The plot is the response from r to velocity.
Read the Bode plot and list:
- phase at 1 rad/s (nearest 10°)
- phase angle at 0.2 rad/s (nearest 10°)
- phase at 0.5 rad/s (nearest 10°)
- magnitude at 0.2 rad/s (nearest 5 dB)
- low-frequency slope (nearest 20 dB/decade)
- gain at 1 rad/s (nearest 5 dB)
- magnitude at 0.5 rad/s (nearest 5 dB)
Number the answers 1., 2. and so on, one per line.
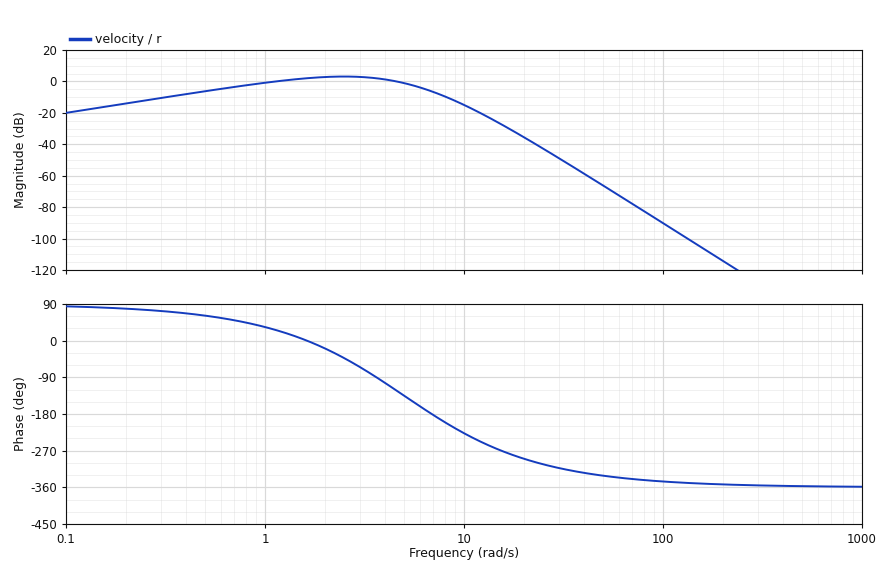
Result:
1. 30°
2. 80°
3. 60°
4. -15 dB
5. 20 dB/decade
6. 0 dB
7. -5 dB
